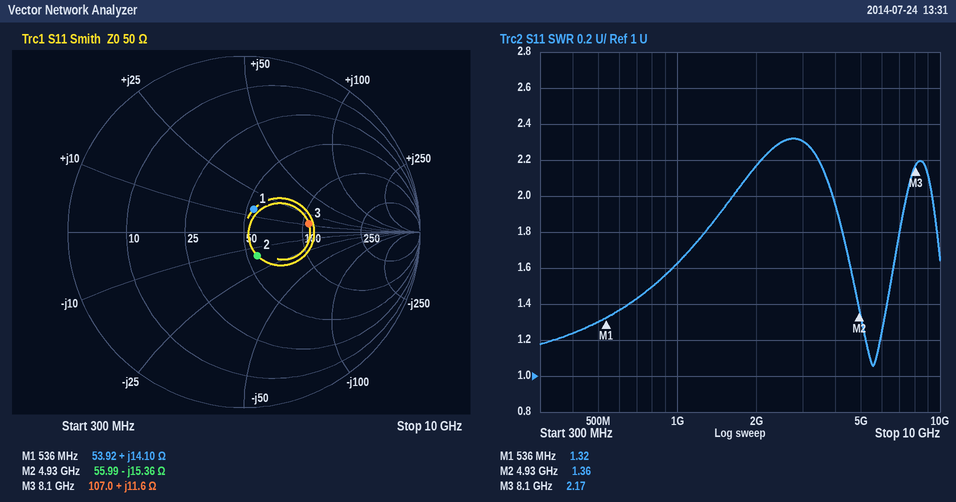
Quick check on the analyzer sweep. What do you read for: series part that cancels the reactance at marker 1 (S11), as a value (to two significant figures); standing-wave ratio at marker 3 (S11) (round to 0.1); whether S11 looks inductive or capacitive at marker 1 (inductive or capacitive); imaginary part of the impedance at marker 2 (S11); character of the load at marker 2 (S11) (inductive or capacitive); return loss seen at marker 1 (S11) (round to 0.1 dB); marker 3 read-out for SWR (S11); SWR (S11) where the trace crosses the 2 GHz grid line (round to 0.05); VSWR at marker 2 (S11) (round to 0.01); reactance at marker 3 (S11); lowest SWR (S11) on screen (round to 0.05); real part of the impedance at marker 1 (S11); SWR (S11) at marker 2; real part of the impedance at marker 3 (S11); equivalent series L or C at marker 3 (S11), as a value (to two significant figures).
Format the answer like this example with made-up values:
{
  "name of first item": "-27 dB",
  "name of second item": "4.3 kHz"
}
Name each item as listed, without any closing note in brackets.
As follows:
{
  "series part that cancels the reactance at marker 1 (S11), as a value": "21 pF",
  "standing-wave ratio at marker 3 (S11)": "2.2",
  "whether S11 looks inductive or capacitive at marker 1": "inductive",
  "imaginary part of the impedance at marker 2": "-15.36 Ω",
  "character of the load at marker 2 (S11)": "capacitive",
  "return loss seen at marker 1 (S11)": "17.1 dB",
  "marker 3 read-out for SWR": "2.17",
  "SWR (S11) where the trace crosses the 2 GHz grid line": "2.15",
  "VSWR at marker 2 (S11)": "1.36",
  "reactance at marker 3": "+11.6 Ω",
  "lowest SWR (S11) on screen": "1.05",
  "real part of the impedance at marker 1": "53.92 Ω",
  "SWR (S11) at marker 2": "1.36",
  "real part of the impedance at marker 3": "107.0 Ω",
  "equivalent series L or C at marker 3 (S11), as a value": "230 pH"
}
